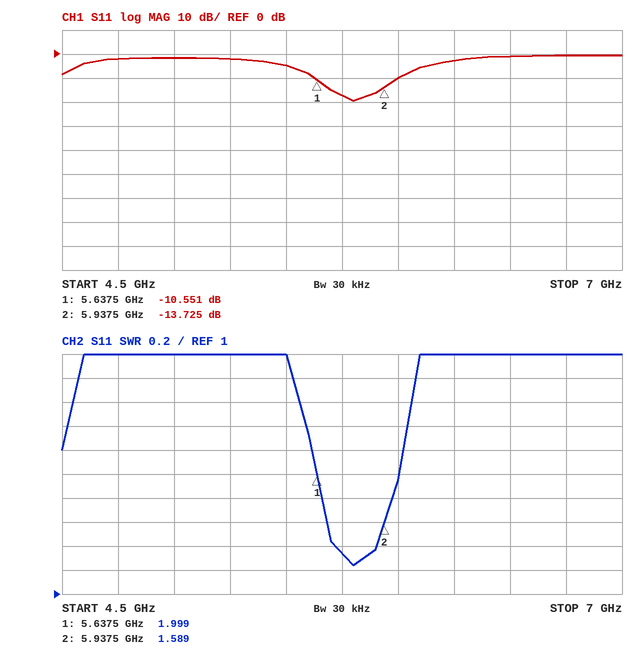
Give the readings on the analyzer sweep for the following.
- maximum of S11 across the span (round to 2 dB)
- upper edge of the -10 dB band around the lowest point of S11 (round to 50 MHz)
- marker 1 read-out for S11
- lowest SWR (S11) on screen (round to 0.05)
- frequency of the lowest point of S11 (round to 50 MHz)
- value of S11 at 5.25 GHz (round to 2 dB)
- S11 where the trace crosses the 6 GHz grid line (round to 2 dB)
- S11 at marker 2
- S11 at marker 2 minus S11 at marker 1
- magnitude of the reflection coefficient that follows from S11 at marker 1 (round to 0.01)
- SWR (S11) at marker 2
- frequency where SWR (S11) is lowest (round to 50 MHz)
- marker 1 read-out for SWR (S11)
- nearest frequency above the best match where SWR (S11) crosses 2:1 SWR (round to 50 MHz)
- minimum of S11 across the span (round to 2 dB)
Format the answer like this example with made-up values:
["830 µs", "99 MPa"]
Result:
["0 dB", "6.00 GHz", "-10.551 dB", "1.25", "5.80 GHz", "-2 dB", "-10 dB", "-13.725 dB", "-3.174 dB", "0.30", "1.589", "5.80 GHz", "1.999", "6.00 GHz", "-20 dB"]
